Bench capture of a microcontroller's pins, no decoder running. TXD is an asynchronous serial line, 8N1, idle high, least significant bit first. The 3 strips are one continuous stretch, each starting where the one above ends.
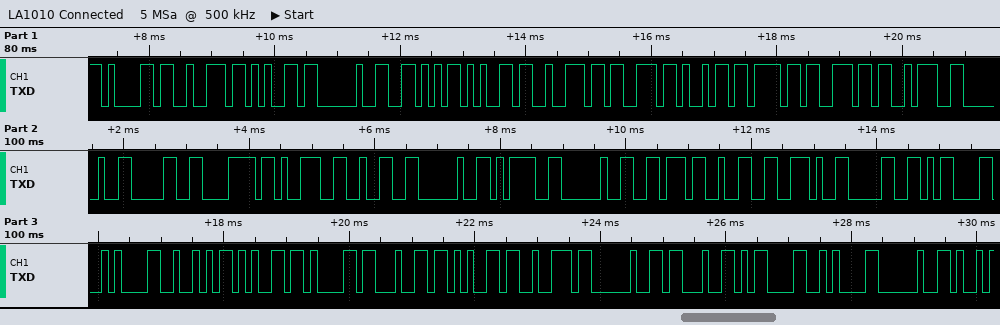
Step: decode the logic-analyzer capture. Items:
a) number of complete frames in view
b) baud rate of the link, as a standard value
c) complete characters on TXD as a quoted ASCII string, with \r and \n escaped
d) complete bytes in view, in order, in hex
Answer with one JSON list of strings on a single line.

["37", "9600 baud", "\"are Version: 0x92 = v2.0\\r\\nReader #\\r\\n \"", "61 72 65 20 56 65 72 73 69 6F 6E 3A 20 30 78 39 32 20 3D 20 76 32 2E 30 0D 0A 52 65 61 64 65 72 20 23 0D 0A 20"]
